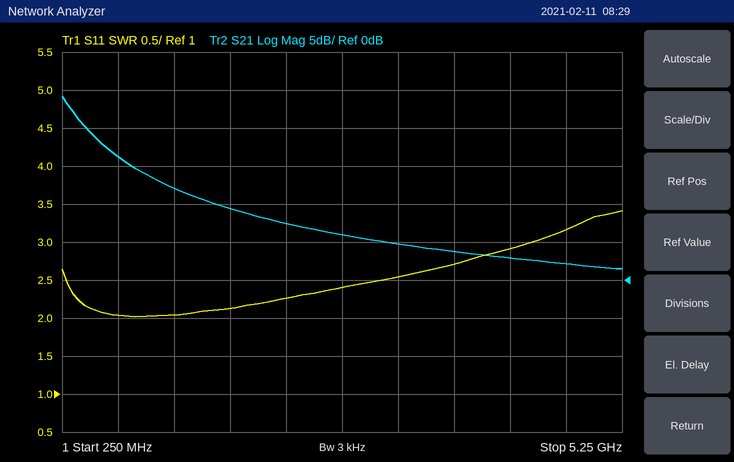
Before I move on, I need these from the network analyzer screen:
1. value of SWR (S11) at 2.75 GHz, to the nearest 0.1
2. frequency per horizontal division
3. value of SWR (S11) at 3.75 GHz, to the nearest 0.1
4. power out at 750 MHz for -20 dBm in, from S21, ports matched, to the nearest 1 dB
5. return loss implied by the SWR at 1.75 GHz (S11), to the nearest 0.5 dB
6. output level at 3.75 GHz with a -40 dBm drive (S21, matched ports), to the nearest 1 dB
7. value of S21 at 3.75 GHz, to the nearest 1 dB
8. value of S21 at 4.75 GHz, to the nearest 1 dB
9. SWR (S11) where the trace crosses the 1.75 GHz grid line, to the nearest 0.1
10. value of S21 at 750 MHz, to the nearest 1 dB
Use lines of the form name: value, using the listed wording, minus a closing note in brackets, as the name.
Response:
value of SWR (S11) at 2.75 GHz, to the nearest 0.1: 2.4
frequency per horizontal division: 500 MHz
value of SWR (S11) at 3.75 GHz, to the nearest 0.1: 2.7
power out at 750 MHz for -20 dBm in, from S21, ports matched, to the nearest 1 dB: -4 dBm
return loss implied by the SWR at 1.75 GHz (S11), to the nearest 0.5 dB: 9.0 dB
output level at 3.75 GHz with a -40 dBm drive (S21, matched ports), to the nearest 1 dB: -36 dBm
value of S21 at 3.75 GHz, to the nearest 1 dB: 4 dB
value of S21 at 4.75 GHz, to the nearest 1 dB: 2 dB
SWR (S11) where the trace crosses the 1.75 GHz grid line, to the nearest 0.1: 2.1
value of S21 at 750 MHz, to the nearest 1 dB: 16 dB
